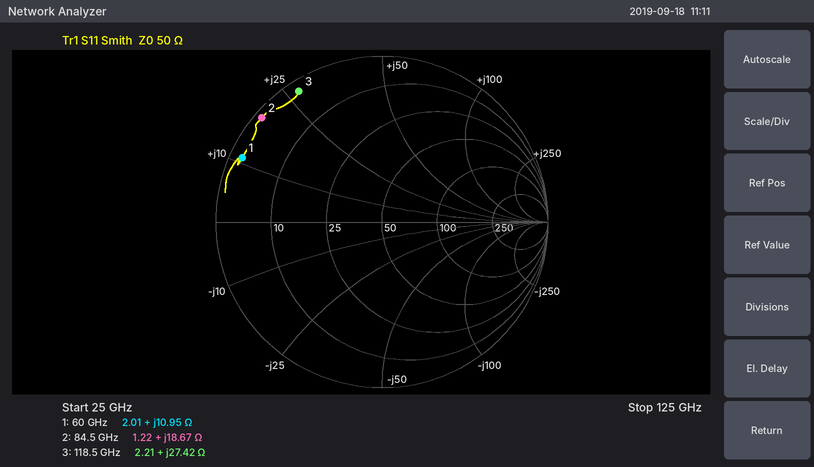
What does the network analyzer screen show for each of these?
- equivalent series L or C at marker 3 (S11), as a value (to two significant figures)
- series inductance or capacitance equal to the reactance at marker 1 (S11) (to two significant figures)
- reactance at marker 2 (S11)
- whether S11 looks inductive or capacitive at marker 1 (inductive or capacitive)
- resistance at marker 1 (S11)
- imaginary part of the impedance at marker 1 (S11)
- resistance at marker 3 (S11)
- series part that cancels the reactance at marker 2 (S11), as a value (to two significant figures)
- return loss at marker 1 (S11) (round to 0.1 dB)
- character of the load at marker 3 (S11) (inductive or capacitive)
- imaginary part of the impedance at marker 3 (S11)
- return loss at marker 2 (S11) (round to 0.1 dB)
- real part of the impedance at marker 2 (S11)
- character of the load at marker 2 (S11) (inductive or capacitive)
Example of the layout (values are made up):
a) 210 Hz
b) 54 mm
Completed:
a) 37 pH
b) 29 pH
c) +18.67 Ω
d) inductive
e) 2.01 Ω
f) +10.95 Ω
g) 2.21 Ω
h) 100 fF
i) 0.7 dB
j) inductive
k) +27.42 Ω
l) 0.4 dB
m) 1.22 Ω
n) inductive
